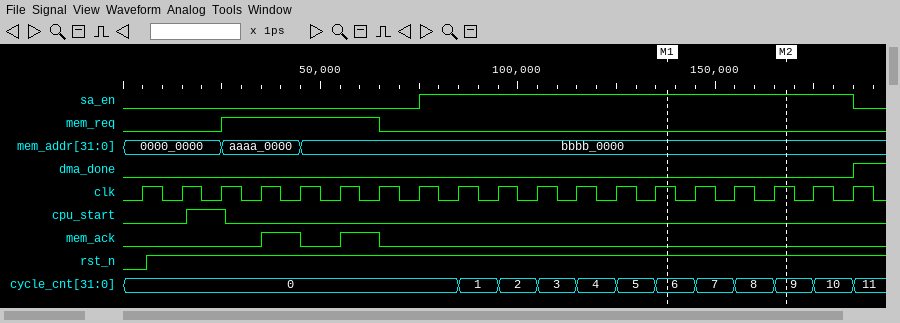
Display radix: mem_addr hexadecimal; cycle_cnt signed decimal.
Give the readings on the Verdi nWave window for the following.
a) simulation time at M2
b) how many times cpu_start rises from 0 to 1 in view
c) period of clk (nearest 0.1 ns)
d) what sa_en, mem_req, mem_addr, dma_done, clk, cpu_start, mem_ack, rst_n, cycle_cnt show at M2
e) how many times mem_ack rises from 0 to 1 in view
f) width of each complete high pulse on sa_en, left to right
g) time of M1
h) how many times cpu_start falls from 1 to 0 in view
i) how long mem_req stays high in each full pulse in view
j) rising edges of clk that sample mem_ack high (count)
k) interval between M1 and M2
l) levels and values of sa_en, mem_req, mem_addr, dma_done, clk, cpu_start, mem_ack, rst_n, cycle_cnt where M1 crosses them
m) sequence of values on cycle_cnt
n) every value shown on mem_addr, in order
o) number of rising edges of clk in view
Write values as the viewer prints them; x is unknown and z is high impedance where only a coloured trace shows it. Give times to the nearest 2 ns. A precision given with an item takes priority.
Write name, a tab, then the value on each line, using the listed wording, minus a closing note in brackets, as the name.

simulation time at M2	168 ns
how many times cpu_start rises from 0 to 1 in view	1
period of clk	10 ns
what sa_en, mem_req, mem_addr, dma_done, clk, cpu_start, mem_ack, rst_n, cycle_cnt show at M2	sa_en=1, mem_req=0, mem_addr=bbbb_0000, dma_done=0, clk=1, cpu_start=0, mem_ack=0, rst_n=1, cycle_cnt=9
how many times mem_ack rises from 0 to 1 in view	2
width of each complete high pulse on sa_en, left to right	110 ns
time of M1	138 ns
how many times cpu_start falls from 1 to 0 in view	1
how long mem_req stays high in each full pulse in view	40 ns
rising edges of clk that sample mem_ack high	2
interval between M1 and M2	30 ns
levels and values of sa_en, mem_req, mem_addr, dma_done, clk, cpu_start, mem_ack, rst_n, cycle_cnt where M1 crosses them	sa_en=1, mem_req=0, mem_addr=bbbb_0000, dma_done=0, clk=1, cpu_start=0, mem_ack=0, rst_n=1, cycle_cnt=6
sequence of values on cycle_cnt	0, 1, 2, 3, 4, 5, 6, 7, 8, 9, 10, 11
every value shown on mem_addr, in order	0000_0000, aaaa_0000, bbbb_0000
number of rising edges of clk in view	19
